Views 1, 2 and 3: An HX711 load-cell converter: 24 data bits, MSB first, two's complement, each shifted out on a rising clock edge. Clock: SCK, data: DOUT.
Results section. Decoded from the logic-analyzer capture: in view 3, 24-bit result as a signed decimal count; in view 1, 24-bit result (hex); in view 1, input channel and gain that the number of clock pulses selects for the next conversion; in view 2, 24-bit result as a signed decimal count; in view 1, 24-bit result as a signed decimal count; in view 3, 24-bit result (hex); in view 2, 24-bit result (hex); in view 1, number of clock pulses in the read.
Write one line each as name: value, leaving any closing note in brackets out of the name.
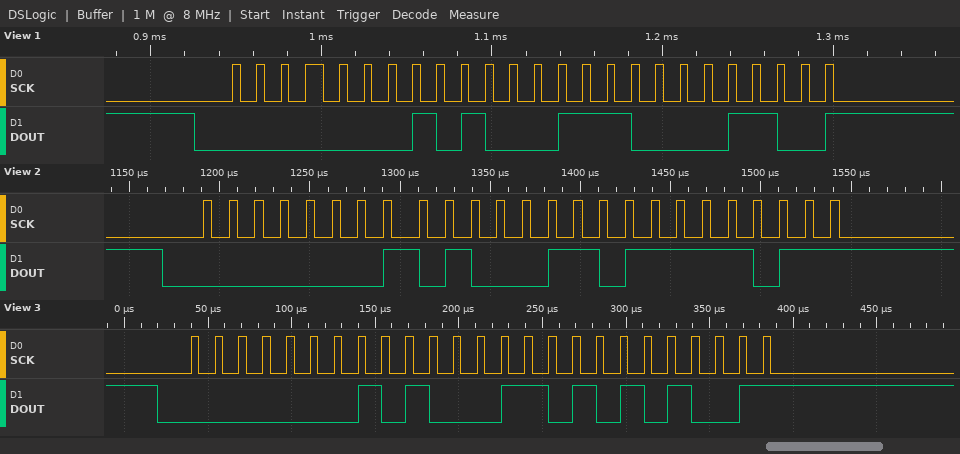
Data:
in view 3, 24-bit result as a signed decimal count: 83625
in view 1, 24-bit result: 0x01470C
in view 1, input channel and gain that the number of clock pulses selects for the next conversion: channel A, gain 128
in view 2, 24-bit result as a signed decimal count: 83707
in view 1, 24-bit result as a signed decimal count: 83724
in view 3, 24-bit result: 0x0146A9
in view 2, 24-bit result: 0x0146FB
in view 1, number of clock pulses in the read: 25
